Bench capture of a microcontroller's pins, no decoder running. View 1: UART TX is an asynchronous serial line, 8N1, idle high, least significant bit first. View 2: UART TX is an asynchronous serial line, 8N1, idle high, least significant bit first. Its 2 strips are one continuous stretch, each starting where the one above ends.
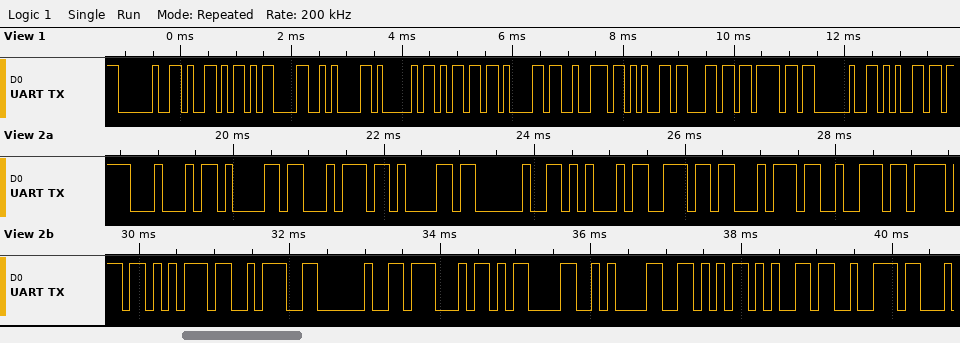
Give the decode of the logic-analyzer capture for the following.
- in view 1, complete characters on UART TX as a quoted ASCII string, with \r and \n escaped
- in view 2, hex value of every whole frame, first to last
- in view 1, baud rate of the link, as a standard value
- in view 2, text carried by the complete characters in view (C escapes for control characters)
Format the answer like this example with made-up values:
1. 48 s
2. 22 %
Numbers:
1. " Y\r\nAmarelo e"
2. 44 61 74 61 20 45 6E 74 72 6F 75 3A 20 47 0D 0A 56 65 72
3. 9600 baud
4. "Data Entrou: G\r\nVer"
